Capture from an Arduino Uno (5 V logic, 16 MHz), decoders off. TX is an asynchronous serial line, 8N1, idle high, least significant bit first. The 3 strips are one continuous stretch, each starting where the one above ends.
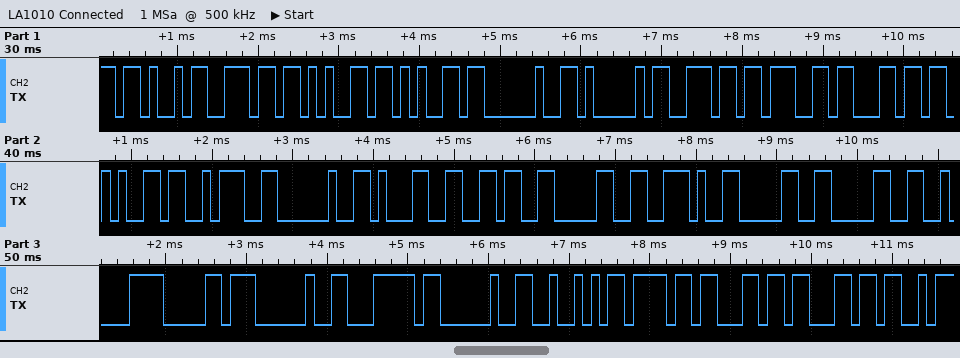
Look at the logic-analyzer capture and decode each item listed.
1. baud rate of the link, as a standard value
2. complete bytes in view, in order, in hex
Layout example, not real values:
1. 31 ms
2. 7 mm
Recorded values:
1. 9600 baud
2. 4B 6E 65 65 20 41 6E 67 6C 65 3A 20 31 36 30 2E 30 30 C2 B0 20 7C 20 52 6F 6C 6C
